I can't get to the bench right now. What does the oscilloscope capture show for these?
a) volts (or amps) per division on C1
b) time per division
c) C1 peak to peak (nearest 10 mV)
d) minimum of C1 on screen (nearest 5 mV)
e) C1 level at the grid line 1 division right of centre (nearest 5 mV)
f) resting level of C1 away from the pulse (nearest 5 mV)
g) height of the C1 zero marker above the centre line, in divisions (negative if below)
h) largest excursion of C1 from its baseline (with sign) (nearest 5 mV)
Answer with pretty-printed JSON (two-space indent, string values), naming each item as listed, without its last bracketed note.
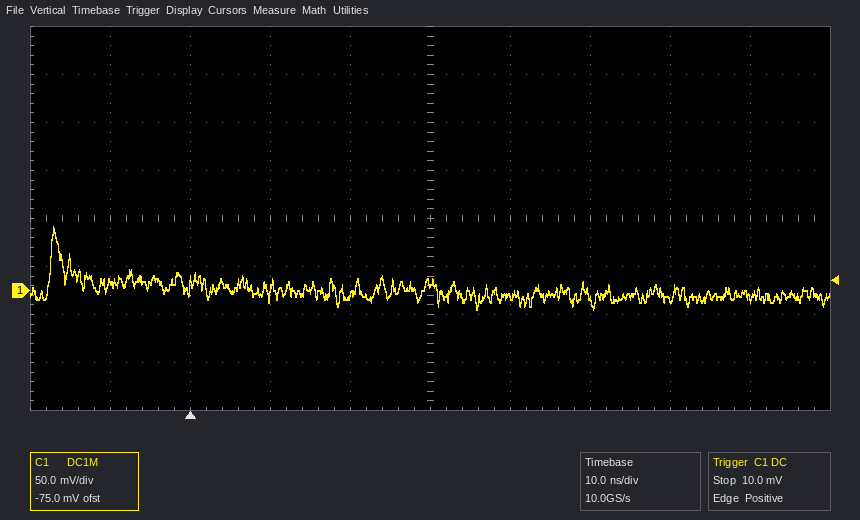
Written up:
{
  "volts (or amps) per division on C1": "50 mV",
  "time per division": "10 ns",
  "C1 peak to peak": "90 mV",
  "minimum of C1 on screen": "-20 mV",
  "C1 level at the grid line 1 division right of centre": "-5 mV",
  "resting level of C1 away from the pulse": "-5 mV",
  "height of the C1 zero marker above the centre line, in divisions": "-1.5 div",
  "largest excursion of C1 from its baseline (with sign)": "+70 mV"
}
